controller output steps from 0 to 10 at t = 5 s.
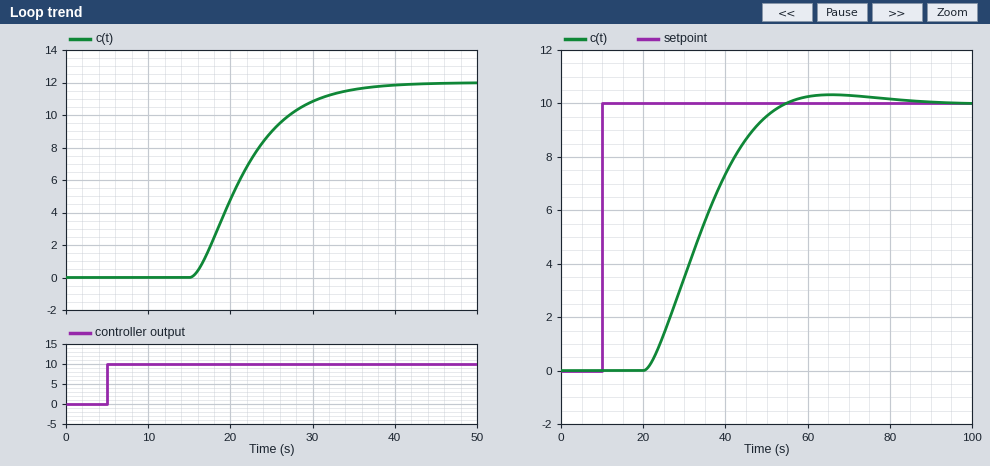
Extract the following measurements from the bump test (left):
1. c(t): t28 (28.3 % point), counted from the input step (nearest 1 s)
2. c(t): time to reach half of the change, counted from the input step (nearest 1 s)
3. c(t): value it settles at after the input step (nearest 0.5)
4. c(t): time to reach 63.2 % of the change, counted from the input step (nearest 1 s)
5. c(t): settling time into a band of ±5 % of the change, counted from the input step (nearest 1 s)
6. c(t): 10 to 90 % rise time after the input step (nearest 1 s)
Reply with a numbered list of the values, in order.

1. 14 s
2. 16 s
3. 12.0
4. 18 s
5. 28 s
6. 13 s
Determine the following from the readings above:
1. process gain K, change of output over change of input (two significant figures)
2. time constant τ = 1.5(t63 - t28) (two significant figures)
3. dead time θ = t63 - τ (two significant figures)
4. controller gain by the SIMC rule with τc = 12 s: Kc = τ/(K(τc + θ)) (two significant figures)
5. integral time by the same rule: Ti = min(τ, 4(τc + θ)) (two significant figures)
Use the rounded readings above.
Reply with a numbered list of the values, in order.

1. 1.2
2. 6.0 s
3. 12 s
4. 0.21
5. 6.0 s
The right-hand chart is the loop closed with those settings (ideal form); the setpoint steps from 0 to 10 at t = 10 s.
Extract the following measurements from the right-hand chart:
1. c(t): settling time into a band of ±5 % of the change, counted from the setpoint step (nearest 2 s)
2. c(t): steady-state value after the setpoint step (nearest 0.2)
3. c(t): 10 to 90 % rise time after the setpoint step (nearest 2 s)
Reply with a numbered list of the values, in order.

1. 40 s
2. 10.0
3. 22 s
